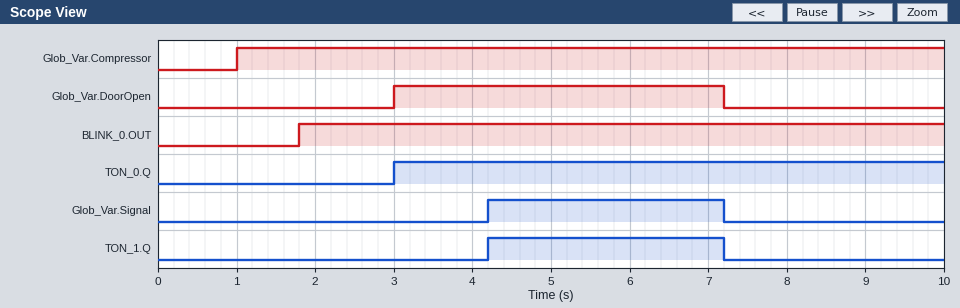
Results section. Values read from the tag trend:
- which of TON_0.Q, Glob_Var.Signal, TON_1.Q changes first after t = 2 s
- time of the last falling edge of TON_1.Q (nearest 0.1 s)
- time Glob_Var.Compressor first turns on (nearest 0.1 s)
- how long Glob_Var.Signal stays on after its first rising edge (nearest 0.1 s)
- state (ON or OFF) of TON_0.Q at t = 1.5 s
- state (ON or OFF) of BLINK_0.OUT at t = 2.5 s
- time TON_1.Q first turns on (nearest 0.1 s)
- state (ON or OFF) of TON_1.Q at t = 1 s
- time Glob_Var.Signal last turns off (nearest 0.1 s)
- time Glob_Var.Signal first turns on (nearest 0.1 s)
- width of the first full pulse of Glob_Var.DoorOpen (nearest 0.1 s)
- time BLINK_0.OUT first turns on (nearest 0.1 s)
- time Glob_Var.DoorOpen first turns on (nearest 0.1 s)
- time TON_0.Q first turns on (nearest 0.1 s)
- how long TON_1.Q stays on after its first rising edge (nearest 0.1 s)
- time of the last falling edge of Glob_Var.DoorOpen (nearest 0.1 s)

TON_0.Q
7.2 s
1.0 s
3.0 s
OFF
ON
4.2 s
OFF
7.2 s
4.2 s
4.2 s
1.8 s
3.0 s
3.0 s
3.0 s
7.2 s
